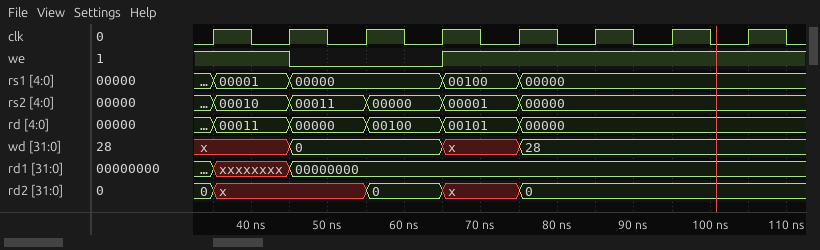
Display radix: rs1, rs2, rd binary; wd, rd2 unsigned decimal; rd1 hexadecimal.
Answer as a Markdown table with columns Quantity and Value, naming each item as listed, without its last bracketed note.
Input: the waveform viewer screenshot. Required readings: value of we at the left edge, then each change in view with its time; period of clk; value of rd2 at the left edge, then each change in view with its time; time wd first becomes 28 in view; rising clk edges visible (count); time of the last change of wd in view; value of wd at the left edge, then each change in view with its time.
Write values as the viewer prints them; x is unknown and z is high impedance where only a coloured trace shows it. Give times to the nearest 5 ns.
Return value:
| Quantity | Value |
|---|---|
| value of we at the left edge, then each change in view with its time | 1, 0 at 45 ns, 1 at 65 ns |
| period of clk | 10 ns |
| value of rd2 at the left edge, then each change in view with its time | 0, x at 35 ns, 0 at 55 ns, x at 65 ns, 0 at 75 ns |
| time wd first becomes 28 in view | 75 ns |
| rising clk edges visible | 8 |
| time of the last change of wd in view | 75 ns |
| value of wd at the left edge, then each change in view with its time | x, 0 at 45 ns, x at 65 ns, 28 at 75 ns |
